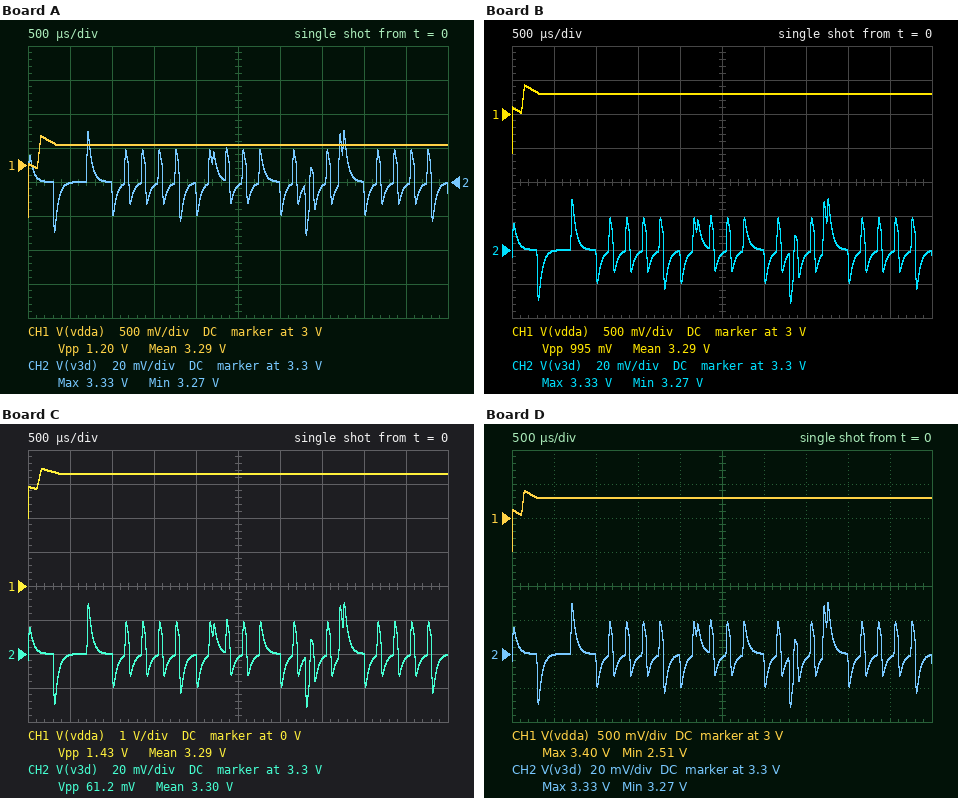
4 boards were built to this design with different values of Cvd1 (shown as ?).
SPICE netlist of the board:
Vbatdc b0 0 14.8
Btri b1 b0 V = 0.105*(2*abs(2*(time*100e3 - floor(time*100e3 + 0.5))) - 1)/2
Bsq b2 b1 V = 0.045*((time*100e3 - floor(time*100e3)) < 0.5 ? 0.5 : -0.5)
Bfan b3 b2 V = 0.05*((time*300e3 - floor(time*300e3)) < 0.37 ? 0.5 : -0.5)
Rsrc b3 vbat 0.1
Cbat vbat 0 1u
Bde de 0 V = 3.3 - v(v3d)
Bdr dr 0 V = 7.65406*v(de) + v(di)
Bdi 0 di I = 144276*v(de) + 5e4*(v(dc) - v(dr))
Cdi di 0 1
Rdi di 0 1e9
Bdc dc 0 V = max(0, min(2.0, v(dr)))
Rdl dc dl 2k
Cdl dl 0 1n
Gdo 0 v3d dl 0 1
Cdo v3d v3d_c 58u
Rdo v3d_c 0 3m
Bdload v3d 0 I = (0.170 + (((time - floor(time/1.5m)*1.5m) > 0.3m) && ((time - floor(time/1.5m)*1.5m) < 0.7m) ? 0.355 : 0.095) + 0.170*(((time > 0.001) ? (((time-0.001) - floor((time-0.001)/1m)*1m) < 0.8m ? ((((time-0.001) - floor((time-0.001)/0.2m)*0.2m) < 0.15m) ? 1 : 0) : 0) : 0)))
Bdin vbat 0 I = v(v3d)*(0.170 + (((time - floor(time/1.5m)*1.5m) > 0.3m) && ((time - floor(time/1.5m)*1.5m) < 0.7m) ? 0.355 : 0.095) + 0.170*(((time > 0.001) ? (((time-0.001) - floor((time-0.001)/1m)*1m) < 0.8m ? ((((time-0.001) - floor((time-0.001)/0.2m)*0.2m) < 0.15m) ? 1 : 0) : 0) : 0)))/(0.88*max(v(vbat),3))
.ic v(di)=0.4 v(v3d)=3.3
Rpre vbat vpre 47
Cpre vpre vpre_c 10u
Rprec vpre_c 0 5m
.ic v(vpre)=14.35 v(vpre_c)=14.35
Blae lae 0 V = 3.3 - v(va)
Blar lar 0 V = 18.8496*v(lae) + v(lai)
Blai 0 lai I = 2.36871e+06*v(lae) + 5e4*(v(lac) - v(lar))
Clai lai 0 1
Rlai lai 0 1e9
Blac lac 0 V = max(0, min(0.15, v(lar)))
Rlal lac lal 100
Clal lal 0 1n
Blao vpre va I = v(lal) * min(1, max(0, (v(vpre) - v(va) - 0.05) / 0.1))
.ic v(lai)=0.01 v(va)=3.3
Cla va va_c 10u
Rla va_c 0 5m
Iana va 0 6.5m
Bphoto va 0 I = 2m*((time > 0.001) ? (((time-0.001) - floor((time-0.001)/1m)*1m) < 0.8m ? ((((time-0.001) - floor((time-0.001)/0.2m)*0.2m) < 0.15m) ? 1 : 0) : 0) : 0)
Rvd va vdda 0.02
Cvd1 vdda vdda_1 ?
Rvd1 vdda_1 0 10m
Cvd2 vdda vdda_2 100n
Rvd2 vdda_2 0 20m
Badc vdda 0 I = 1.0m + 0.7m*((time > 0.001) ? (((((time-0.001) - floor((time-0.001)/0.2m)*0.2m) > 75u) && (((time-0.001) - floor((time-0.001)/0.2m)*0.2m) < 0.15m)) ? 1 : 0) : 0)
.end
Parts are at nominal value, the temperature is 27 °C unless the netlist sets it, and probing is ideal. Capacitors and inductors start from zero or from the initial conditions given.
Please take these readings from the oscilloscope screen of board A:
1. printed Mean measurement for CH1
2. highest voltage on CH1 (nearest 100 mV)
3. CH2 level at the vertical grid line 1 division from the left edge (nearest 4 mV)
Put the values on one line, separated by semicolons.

3.29 V; 3.4 V; 3.300 V
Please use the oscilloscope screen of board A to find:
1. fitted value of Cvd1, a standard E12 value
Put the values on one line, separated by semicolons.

820 nF
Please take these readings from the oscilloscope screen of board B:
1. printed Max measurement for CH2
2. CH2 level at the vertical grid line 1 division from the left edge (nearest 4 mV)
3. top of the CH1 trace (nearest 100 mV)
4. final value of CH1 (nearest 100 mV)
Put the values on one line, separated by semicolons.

3.33 V; 3.300 V; 3.4 V; 3.3 V
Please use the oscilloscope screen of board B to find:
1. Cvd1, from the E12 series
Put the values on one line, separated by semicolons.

560 nF
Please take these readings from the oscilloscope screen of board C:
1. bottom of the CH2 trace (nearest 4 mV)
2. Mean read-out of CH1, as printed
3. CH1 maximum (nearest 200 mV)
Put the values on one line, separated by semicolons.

3.268 V; 3.29 V; 3.4 V
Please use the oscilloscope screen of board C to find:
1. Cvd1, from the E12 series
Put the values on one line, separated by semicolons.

1.2 µF
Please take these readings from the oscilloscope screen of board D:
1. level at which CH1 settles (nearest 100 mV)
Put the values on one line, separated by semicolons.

3.3 V
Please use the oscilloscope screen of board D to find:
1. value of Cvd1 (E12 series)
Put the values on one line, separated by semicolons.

470 nF
